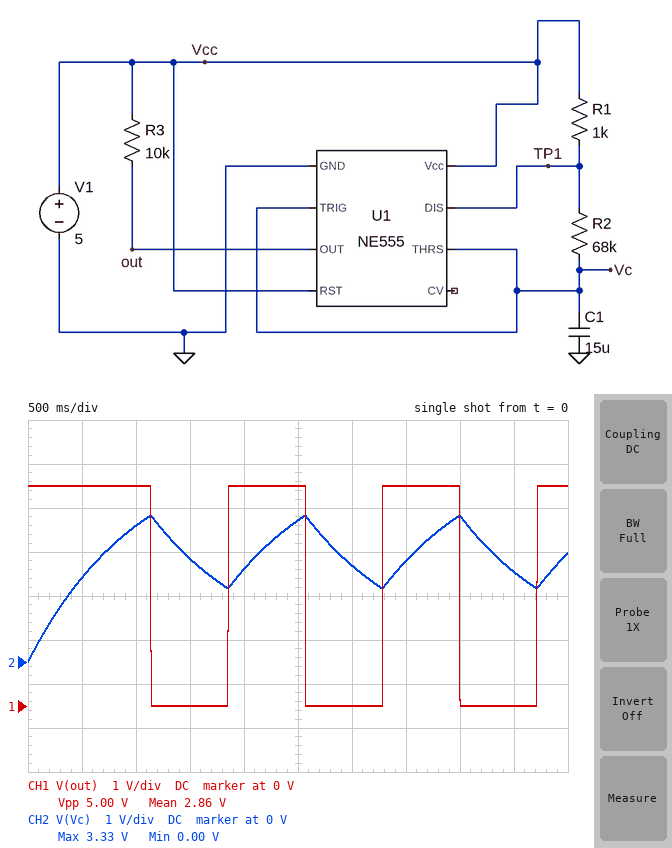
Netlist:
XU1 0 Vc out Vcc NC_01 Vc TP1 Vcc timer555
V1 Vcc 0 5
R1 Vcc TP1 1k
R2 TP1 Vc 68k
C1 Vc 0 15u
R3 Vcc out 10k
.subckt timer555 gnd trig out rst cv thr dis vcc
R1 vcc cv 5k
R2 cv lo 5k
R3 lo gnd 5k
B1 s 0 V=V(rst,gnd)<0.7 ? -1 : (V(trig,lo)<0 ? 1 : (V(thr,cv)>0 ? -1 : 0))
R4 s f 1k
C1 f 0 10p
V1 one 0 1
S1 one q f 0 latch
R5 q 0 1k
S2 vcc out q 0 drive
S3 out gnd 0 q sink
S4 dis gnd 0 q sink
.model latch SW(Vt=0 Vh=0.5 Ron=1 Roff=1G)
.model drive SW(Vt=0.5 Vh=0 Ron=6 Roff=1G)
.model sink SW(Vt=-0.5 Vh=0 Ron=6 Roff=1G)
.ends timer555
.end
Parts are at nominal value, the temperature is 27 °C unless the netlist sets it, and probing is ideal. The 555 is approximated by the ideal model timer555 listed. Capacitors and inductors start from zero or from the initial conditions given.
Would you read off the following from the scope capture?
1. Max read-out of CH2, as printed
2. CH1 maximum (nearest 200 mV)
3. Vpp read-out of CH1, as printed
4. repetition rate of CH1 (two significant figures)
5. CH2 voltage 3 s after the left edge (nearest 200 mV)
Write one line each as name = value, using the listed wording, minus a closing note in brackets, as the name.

Max read-out of CH2, as printed = 3.33 V
CH1 maximum = 5.0 V
Vpp read-out of CH1, as printed = 5.00 V
repetition rate of CH1 = 700 mHz
CH2 voltage 3 s after the left edge = 2.2 V
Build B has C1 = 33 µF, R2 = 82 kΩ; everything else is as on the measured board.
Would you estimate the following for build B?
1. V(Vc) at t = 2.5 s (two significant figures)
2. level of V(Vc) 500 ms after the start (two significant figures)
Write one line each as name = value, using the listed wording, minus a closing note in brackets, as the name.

V(Vc) at t = 2.5 s = 3.0 V
level of V(Vc) 500 ms after the start = 830 mV
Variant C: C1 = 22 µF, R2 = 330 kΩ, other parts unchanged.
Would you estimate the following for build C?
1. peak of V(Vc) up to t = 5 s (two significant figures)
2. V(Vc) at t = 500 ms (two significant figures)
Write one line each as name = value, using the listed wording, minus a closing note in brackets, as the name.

peak of V(Vc) up to t = 5 s = 2.5 V
V(Vc) at t = 500 ms = 330 mV
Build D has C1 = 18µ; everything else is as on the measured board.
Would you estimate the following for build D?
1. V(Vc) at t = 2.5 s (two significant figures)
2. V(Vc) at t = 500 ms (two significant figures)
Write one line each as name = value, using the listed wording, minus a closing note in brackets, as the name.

V(Vc) at t = 2.5 s = 2.3 V
V(Vc) at t = 500 ms = 1.7 V
